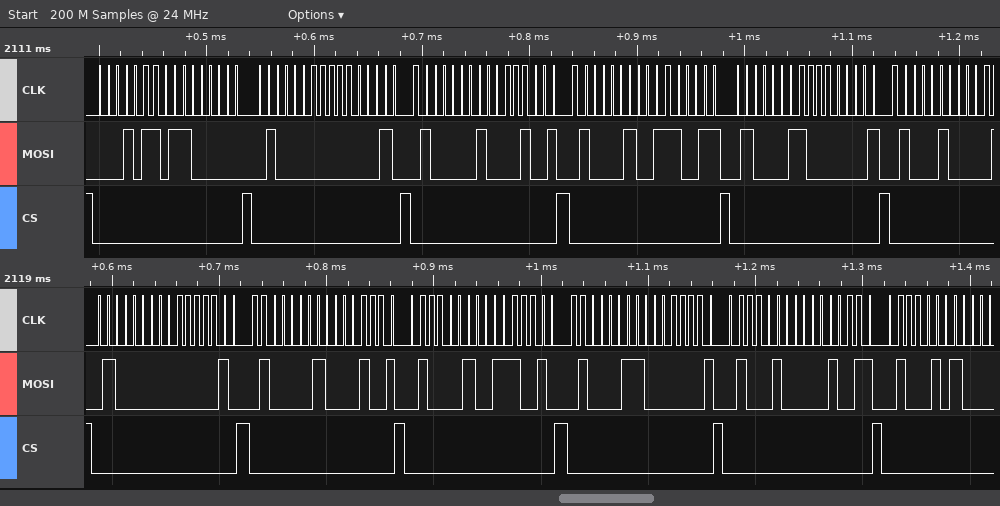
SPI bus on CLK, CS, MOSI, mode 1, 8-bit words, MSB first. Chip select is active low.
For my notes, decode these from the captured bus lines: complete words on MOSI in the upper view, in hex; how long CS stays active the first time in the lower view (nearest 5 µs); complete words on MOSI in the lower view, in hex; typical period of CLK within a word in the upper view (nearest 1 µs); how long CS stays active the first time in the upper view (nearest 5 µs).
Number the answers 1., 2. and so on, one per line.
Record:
1. 16, C0, 40, 02, 41, 09, 42, 73, 43, 01, 44
2. 135 µs
3. 40, 02, 41, 09, 42, 72, 43, 01, 44, 13, 45
4. 8 µs
5. 140 µs
